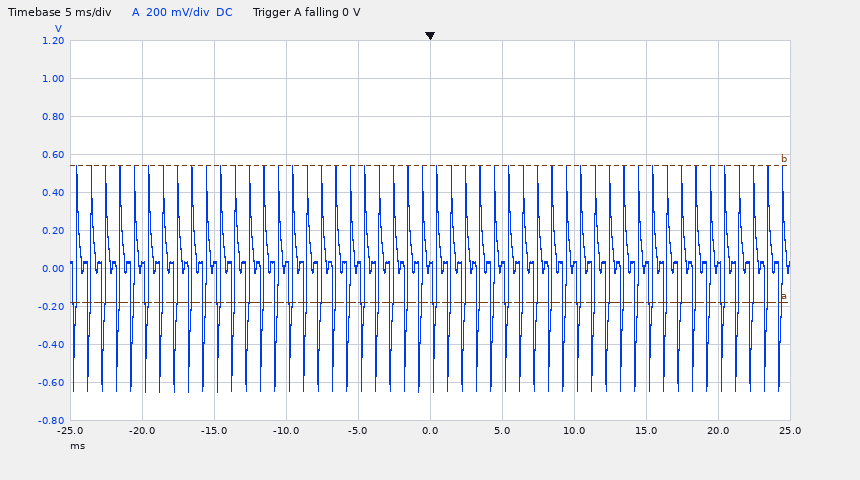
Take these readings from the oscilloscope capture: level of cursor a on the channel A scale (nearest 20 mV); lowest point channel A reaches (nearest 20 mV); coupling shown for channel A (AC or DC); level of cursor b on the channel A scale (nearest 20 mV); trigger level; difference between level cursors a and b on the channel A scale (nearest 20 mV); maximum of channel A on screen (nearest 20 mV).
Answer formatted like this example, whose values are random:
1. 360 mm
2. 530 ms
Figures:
1. -180 mV
2. -640 mV
3. DC
4. 540 mV
5. 0 V
6. 720 mV
7. 540 mV
